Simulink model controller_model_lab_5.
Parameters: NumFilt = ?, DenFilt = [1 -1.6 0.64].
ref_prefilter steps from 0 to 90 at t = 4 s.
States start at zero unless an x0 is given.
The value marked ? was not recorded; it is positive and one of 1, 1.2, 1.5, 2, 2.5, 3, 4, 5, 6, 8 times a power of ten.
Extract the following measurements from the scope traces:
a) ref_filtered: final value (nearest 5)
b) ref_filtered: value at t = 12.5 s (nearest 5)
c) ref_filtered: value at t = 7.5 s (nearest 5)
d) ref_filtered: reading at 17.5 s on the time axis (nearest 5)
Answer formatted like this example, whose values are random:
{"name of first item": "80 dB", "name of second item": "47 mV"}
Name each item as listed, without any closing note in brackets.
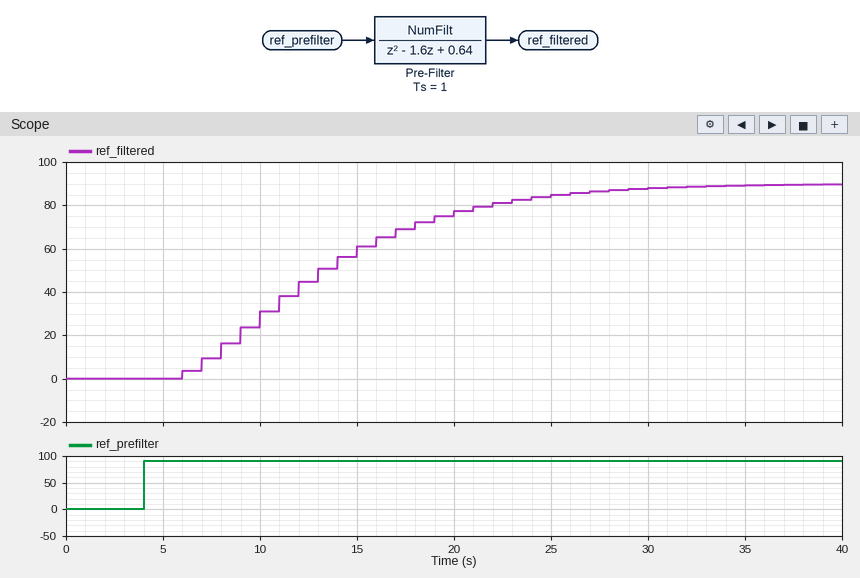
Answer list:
{"ref_filtered: final value": "90", "ref_filtered: value at t = 12.5 s": "45", "ref_filtered: value at t = 7.5 s": "10", "ref_filtered: reading at 17.5 s on the time axis": "70"}
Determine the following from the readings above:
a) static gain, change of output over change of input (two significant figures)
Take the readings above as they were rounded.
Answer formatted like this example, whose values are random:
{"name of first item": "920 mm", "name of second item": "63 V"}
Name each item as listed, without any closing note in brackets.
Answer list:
{"static gain, change of output over change of input": "1.0"}
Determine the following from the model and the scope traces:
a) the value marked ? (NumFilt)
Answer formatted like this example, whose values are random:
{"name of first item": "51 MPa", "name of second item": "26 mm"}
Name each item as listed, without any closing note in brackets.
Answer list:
{"the value marked ?": "0.04"}
